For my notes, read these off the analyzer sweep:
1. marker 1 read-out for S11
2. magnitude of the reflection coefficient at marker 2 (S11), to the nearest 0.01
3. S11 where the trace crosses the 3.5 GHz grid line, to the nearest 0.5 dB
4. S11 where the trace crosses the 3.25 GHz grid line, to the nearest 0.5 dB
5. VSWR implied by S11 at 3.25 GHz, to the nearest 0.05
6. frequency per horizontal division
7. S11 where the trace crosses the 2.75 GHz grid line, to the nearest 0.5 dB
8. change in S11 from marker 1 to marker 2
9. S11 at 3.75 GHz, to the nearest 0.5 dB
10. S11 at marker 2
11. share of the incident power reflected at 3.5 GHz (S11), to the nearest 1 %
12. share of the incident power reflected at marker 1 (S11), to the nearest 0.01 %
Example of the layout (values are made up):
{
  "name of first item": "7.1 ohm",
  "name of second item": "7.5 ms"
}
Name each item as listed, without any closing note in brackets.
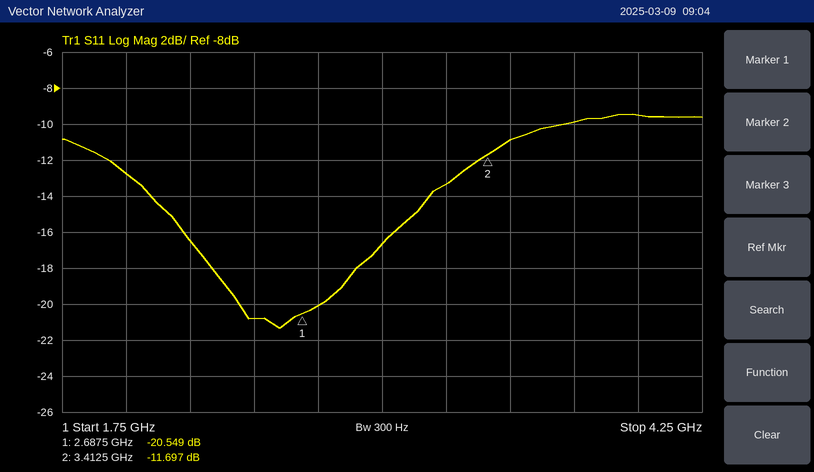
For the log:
{
  "marker 1 read-out for S11": "-20.549 dB",
  "magnitude of the reflection coefficient at marker 2 (S11), to the nearest 0.01": "0.26",
  "S11 where the trace crosses the 3.5 GHz grid line, to the nearest 0.5 dB": "-11.0 dB",
  "S11 where the trace crosses the 3.25 GHz grid line, to the nearest 0.5 dB": "-13.5 dB",
  "VSWR implied by S11 at 3.25 GHz, to the nearest 0.05": "1.55",
  "frequency per horizontal division": "250 MHz",
  "S11 where the trace crosses the 2.75 GHz grid line, to the nearest 0.5 dB": "-20.0 dB",
  "change in S11 from marker 1 to marker 2": "8.852 dB",
  "S11 at 3.75 GHz, to the nearest 0.5 dB": "-10.0 dB",
  "S11 at marker 2": "-11.697 dB",
  "share of the incident power reflected at 3.5 GHz (S11), to the nearest 1 %": "8 %",
  "share of the incident power reflected at marker 1 (S11), to the nearest 0.01 %": "0.88 %"
}
